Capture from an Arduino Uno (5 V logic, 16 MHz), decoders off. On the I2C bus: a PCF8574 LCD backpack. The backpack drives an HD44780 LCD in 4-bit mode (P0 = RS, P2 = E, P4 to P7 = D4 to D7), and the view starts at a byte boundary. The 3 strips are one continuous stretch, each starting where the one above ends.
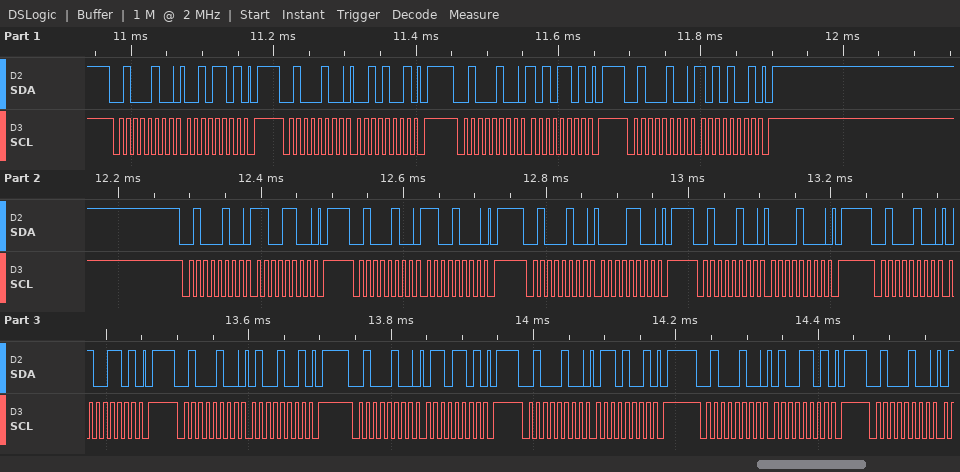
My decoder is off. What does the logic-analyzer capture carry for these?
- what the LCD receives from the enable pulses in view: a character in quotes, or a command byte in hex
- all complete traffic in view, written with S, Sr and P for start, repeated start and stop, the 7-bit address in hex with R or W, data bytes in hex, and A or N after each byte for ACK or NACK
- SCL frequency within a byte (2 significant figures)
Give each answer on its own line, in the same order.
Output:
'*' 0xC0 'F'
S 22W A 2D A P S 22W A 29 A P S 22W A AD A P S 22W A A9 A P S 22W A CC A P S 22W A C8 A P S 22W A 0C A P S 22W A 08 A P S 22W A 4D A P S 22W A 49 A P S 22W A 6D A P S 22W A 69 A P S 22W A 4D A P S 22W A
100 kHz
